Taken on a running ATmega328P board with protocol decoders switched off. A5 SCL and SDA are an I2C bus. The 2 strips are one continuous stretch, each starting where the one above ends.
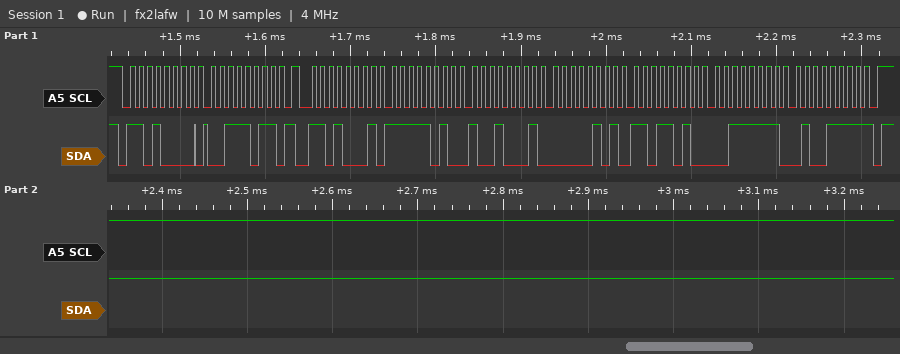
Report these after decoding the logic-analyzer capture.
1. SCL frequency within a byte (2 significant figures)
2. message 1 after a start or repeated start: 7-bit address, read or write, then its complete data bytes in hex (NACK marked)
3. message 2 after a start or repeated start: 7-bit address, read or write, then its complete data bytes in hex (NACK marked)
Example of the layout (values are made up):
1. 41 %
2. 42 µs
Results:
1. 100 kHz
2. 0x68 write: 3B
3. 0x68 read: FA 91 05 DA 3F 4F NACK
